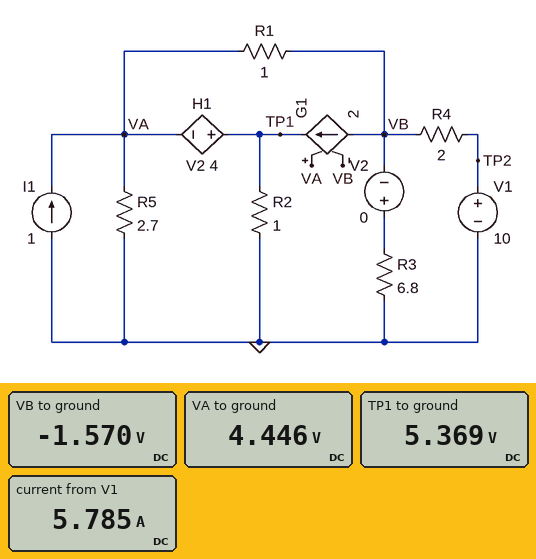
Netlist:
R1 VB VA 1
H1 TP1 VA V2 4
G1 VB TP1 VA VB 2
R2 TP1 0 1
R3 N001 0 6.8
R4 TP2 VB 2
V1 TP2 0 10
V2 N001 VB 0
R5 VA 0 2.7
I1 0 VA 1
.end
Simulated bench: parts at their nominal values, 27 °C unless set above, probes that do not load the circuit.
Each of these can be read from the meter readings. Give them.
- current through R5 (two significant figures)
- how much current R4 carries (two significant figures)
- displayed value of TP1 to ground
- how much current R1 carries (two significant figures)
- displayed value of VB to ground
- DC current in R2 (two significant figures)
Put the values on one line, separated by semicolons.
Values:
1.6 A; 5.8 A; 5.369 V; 6.0 A; -1.570 V; 5.4 A
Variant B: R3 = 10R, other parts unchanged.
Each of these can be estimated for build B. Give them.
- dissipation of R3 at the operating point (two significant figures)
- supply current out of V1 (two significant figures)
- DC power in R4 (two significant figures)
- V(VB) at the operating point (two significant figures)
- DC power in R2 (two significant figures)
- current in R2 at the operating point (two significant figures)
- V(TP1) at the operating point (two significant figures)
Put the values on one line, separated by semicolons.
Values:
130 mW; 5.6 A; 62 W; -1.1 V; 25 W; 5.0 A; 5.0 V
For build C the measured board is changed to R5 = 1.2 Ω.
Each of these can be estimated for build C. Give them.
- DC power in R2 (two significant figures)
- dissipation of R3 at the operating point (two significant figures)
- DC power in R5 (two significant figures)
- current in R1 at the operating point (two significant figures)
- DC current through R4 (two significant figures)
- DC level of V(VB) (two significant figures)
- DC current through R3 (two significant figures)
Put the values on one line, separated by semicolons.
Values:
37 W; 3.0 W; 9.7 W; 7.9 A; 7.2 A; -4.5 V; 660 mA
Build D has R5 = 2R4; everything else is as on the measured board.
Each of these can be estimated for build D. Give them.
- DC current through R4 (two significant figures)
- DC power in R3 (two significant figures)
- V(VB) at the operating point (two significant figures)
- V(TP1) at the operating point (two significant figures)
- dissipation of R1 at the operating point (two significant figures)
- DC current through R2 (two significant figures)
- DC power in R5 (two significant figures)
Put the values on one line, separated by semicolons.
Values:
6.0 A; 550 mW; -1.9 V; 5.5 V; 39 W; 5.5 A; 7.8 W
